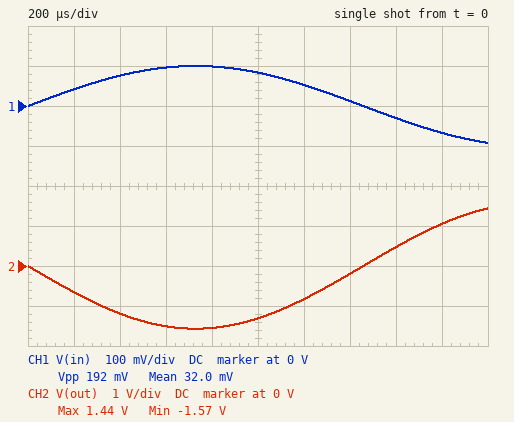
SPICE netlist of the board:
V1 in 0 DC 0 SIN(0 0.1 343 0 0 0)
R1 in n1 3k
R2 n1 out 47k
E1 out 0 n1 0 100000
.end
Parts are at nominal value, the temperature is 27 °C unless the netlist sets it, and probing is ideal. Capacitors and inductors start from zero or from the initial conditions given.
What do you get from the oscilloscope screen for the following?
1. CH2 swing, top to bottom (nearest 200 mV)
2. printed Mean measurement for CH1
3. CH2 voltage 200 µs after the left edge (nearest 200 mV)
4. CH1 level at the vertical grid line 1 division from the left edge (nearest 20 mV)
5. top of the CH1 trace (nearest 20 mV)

3.0 V
32.0 mV
-600 mV
40 mV
100 mV
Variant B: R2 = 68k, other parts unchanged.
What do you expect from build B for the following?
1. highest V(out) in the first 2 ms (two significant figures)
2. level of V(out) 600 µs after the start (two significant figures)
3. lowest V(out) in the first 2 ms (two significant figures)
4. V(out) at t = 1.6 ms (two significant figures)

2.1 V
-2.2 V
-2.3 V
680 mV
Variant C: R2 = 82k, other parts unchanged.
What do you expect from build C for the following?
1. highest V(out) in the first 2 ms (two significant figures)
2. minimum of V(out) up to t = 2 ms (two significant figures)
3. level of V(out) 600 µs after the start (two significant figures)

2.5 V
-2.7 V
-2.6 V
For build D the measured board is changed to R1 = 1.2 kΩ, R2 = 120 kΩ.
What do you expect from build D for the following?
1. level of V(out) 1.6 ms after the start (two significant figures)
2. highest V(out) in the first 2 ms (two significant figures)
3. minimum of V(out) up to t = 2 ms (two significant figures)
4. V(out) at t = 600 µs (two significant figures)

3.0 V
9.2 V
-10 V
-9.6 V
